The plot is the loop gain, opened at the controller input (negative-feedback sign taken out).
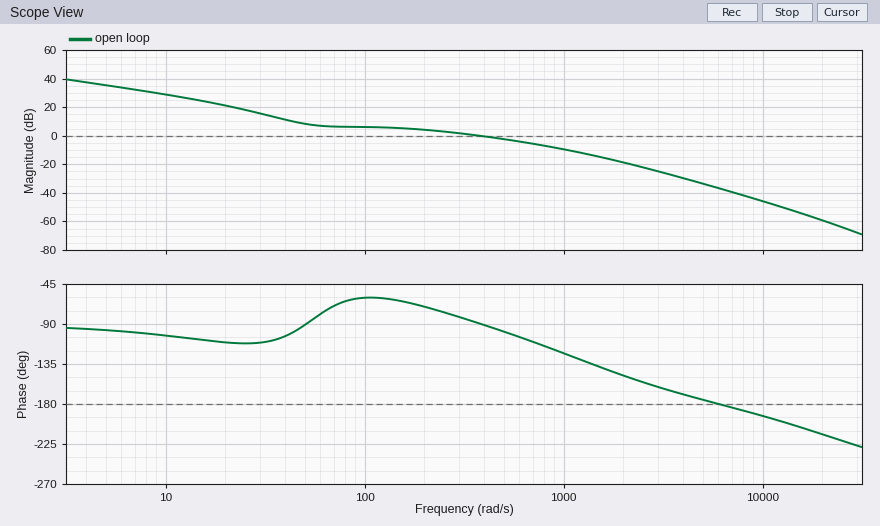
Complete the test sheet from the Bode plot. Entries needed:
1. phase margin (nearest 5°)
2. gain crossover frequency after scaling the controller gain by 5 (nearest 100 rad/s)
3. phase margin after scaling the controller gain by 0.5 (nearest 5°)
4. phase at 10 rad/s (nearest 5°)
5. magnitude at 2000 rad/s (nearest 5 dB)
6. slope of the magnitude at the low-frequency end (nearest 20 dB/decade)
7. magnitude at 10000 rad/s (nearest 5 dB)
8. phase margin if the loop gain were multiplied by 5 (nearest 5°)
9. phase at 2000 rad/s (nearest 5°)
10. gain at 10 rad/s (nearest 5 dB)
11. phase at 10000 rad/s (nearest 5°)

90°
1400 rad/s
120°
-105°
-20 dB
-20 dB/decade
-45 dB
45°
-150°
30 dB
-195°
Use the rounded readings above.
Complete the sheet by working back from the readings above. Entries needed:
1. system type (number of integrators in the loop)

1
